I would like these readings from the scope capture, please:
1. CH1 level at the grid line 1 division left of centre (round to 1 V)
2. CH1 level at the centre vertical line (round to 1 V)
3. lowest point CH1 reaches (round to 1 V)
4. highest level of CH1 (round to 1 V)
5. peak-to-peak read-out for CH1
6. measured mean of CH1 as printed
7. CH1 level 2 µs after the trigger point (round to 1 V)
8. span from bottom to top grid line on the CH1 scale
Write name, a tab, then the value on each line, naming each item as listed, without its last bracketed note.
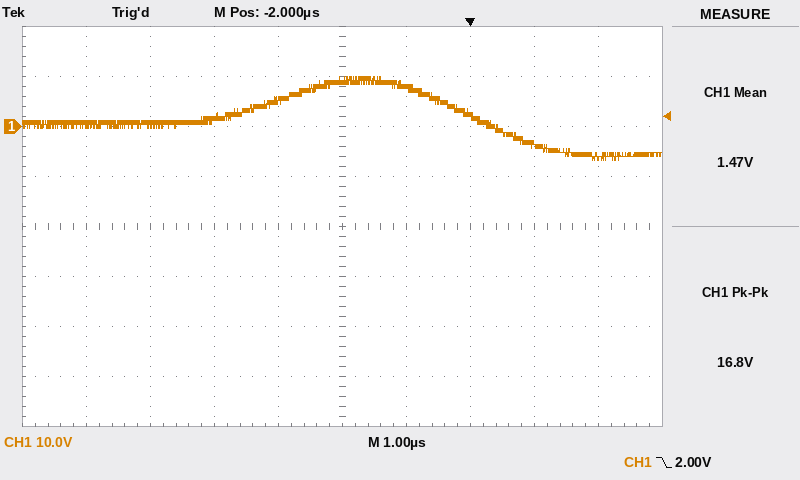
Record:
CH1 level at the grid line 1 division left of centre	5 V
CH1 level at the centre vertical line	9 V
lowest point CH1 reaches	-7 V
highest level of CH1	10 V
peak-to-peak read-out for CH1	16.8 V
measured mean of CH1 as printed	1.47 V
CH1 level 2 µs after the trigger point	-6 V
span from bottom to top grid line on the CH1 scale	80 V
